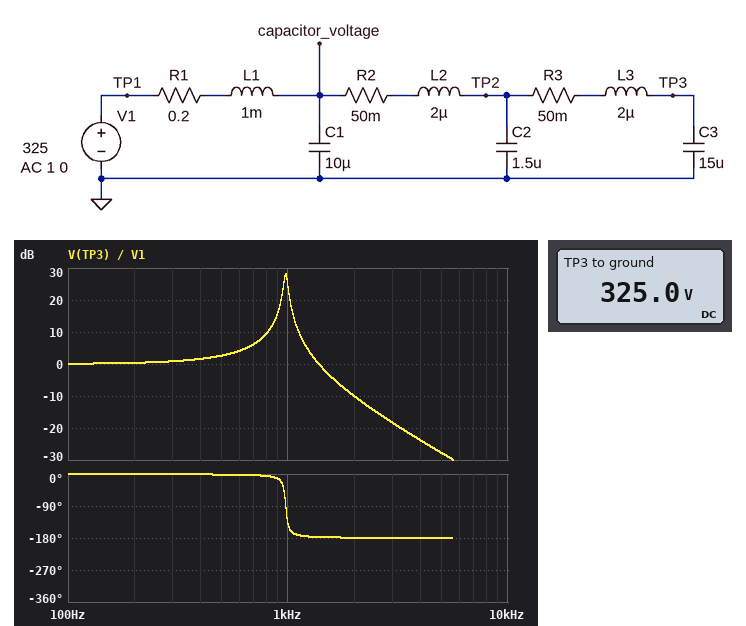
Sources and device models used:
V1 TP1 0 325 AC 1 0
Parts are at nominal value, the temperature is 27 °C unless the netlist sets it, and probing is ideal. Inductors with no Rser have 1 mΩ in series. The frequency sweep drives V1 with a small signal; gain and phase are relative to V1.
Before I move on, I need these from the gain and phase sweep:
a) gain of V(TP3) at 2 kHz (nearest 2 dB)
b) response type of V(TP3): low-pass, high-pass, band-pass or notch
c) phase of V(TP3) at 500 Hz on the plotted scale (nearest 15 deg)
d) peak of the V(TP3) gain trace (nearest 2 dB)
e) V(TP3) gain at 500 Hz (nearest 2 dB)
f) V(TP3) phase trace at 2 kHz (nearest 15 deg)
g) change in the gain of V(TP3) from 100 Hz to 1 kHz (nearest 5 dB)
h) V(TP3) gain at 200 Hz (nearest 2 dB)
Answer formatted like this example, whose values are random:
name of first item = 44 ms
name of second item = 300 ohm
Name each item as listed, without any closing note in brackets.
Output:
gain of V(TP3) at 2 kHz = -10 dB
response type of V(TP3): low-pass, high-pass, band-pass or notch = low-pass
phase of V(TP3) at 500 Hz on the plotted scale = 0 deg
peak of the V(TP3) gain trace = 28 dB
V(TP3) gain at 500 Hz = 2 dB
V(TP3) phase trace at 2 kHz = -180 deg
change in the gain of V(TP3) from 100 Hz to 1 kHz = 25 dB
V(TP3) gain at 200 Hz = 0 dB
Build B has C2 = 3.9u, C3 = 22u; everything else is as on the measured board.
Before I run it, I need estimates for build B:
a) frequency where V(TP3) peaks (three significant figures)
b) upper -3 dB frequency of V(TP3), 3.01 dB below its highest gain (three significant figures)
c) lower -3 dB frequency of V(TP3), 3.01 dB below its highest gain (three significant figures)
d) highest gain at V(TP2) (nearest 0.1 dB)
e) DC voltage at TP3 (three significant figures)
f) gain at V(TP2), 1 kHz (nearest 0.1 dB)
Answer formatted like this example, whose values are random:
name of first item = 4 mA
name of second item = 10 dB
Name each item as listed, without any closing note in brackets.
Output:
frequency where V(TP3) peaks = 839 Hz
upper -3 dB frequency of V(TP3), 3.01 dB below its highest gain = 858 Hz
lower -3 dB frequency of V(TP3), 3.01 dB below its highest gain = 819 Hz
highest gain at V(TP2) = 26.6 dB
DC voltage at TP3 = 325 V
gain at V(TP2), 1 kHz = 7.5 dB
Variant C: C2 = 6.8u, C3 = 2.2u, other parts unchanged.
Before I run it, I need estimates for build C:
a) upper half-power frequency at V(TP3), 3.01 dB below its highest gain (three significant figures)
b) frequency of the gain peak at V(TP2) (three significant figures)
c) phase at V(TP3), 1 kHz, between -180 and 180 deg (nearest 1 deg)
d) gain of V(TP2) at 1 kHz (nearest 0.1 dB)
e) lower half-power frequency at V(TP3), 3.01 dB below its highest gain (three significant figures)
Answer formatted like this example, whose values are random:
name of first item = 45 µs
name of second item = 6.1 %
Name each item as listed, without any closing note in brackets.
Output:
upper half-power frequency at V(TP3), 3.01 dB below its highest gain = 1.17 kHz
frequency of the gain peak at V(TP2) = 1.15 kHz
phase at V(TP3), 1 kHz, between -180 and 180 deg = -6 deg
gain of V(TP2) at 1 kHz = 12.0 dB
lower half-power frequency at V(TP3), 3.01 dB below its highest gain = 1.14 kHz
